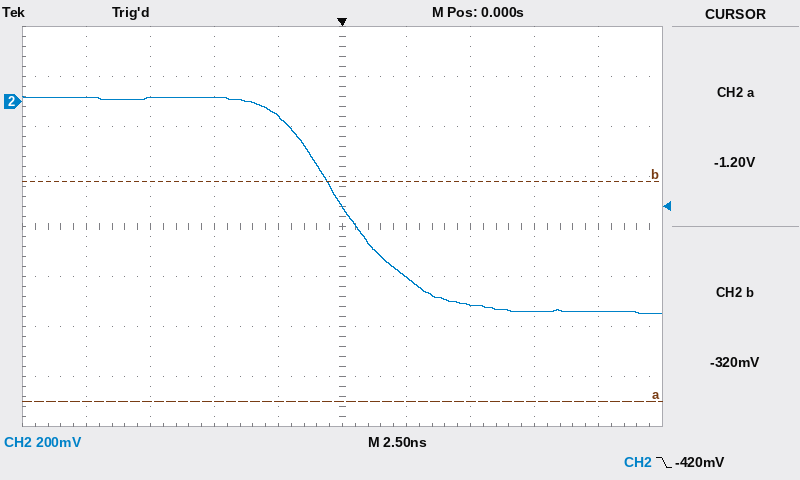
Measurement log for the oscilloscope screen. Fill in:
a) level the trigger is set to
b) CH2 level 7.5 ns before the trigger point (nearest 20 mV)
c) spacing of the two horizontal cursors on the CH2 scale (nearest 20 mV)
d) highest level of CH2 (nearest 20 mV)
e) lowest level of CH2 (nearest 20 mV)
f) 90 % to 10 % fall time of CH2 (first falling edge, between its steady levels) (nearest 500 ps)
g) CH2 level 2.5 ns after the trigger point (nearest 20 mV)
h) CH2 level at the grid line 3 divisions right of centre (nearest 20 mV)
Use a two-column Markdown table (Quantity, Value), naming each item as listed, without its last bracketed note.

| Quantity | Value |
|---|---|
| level the trigger is set to | -420 mV |
| CH2 level 7.5 ns before the trigger point | 20 mV |
| spacing of the two horizontal cursors on the CH2 scale | 880 mV |
| highest level of CH2 | 20 mV |
| lowest level of CH2 | -840 mV |
| 90 % to 10 % fall time of CH2 (first falling edge, between its steady levels) | 5.5 ns |
| CH2 level 2.5 ns after the trigger point | -700 mV |
| CH2 level at the grid line 3 divisions right of centre | -840 mV |
